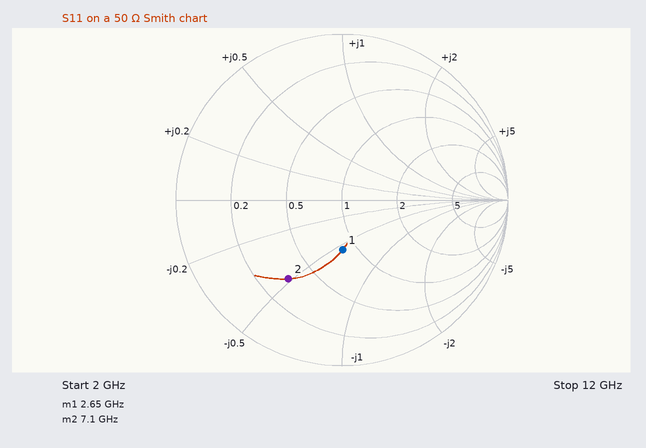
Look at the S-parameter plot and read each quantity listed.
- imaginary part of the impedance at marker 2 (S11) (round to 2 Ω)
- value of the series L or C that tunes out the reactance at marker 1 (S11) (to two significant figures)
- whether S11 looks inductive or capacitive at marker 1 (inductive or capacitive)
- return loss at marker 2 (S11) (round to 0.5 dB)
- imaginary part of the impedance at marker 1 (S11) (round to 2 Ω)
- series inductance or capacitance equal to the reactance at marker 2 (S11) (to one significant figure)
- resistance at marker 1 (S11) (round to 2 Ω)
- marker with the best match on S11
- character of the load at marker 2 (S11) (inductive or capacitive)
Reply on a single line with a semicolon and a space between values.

-24 Ω; 1.7 nH; capacitive; 5.0 dB; -28 Ω; 900 fF; 42 Ω; marker 1; capacitive
